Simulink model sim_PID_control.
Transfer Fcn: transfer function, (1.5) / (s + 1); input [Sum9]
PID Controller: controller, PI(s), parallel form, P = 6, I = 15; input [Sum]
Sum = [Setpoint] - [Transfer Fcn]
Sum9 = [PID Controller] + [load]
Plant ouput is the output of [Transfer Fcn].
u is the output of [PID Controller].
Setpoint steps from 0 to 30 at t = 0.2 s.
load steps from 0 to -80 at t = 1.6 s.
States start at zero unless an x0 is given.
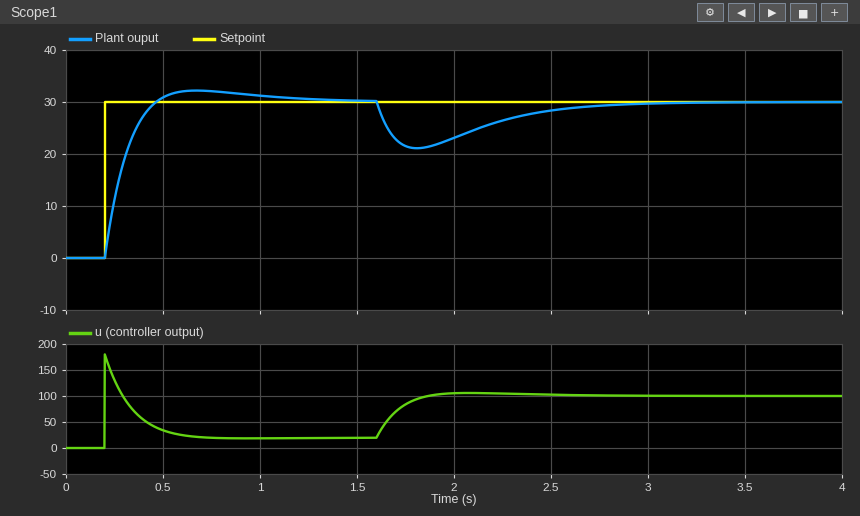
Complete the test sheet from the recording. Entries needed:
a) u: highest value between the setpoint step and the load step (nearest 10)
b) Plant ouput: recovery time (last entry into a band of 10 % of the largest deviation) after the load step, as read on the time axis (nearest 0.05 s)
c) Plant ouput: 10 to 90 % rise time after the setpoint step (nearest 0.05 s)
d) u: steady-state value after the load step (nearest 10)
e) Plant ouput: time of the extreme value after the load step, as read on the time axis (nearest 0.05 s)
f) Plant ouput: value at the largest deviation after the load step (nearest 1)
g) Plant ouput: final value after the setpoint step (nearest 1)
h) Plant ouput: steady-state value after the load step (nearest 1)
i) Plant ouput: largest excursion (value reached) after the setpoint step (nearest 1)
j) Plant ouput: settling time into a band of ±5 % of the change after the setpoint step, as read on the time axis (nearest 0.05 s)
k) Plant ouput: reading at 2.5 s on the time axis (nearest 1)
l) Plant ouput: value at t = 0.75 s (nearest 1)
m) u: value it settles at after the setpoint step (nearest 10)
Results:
180
2.70 s
0.20 s
100
1.80 s
21
30
30
32
0.90 s
28
32
20
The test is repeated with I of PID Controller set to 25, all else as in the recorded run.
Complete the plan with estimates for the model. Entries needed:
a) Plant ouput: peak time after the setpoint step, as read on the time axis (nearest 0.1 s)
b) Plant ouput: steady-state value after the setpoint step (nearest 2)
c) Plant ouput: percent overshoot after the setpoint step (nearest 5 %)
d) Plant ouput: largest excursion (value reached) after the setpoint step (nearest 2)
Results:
0.6 s
30
15 %
34
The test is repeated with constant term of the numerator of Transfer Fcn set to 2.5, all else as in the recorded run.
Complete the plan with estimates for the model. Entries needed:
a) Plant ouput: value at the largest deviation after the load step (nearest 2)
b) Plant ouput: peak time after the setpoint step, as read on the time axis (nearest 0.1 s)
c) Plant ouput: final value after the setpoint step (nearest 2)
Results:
20
0.5 s
30
